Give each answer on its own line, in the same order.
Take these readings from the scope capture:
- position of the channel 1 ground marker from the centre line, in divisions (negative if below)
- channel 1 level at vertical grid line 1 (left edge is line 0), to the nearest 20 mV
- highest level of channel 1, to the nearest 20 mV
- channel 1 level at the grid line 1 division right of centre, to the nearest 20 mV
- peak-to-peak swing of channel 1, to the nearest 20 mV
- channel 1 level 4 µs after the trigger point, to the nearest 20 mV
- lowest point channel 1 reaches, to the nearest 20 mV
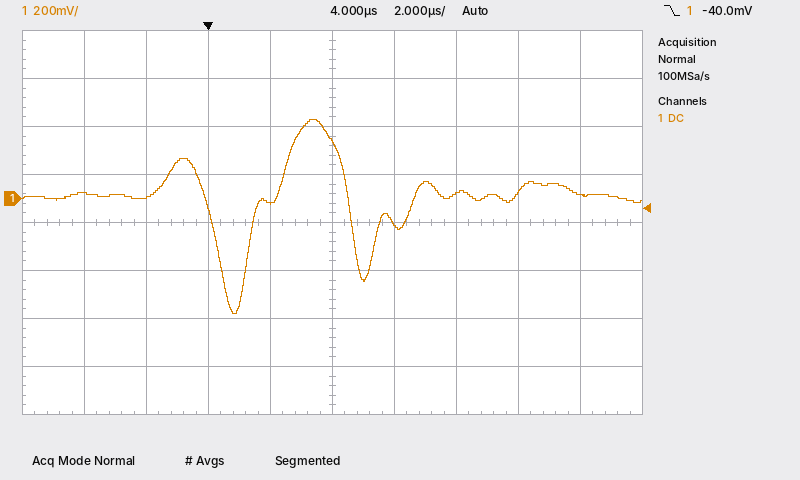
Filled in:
+0.5 div
20 mV
320 mV
-100 mV
800 mV
240 mV
-480 mV
